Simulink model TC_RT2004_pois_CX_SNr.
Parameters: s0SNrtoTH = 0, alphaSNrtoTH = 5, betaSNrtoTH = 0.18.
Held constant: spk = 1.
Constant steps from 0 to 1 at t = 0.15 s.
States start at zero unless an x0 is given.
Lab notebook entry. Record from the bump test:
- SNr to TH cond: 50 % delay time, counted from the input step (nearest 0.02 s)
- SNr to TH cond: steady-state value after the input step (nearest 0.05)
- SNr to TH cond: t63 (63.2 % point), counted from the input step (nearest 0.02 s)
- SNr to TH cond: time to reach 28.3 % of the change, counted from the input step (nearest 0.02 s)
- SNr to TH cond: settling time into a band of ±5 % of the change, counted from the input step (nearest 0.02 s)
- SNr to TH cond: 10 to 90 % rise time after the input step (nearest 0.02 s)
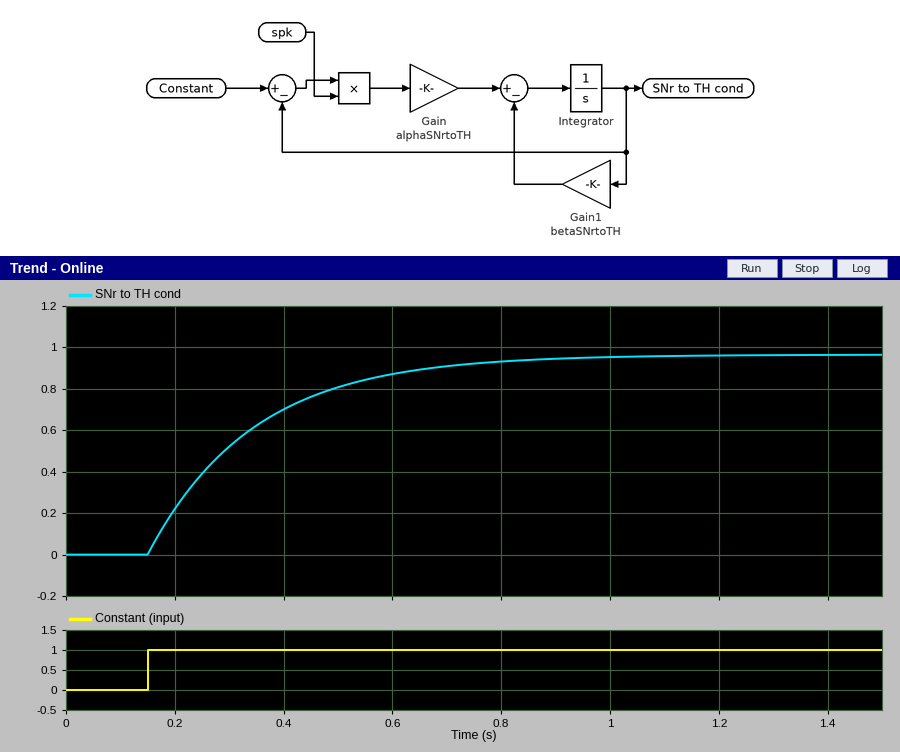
0.14 s
0.95
0.20 s
0.06 s
0.58 s
0.42 s
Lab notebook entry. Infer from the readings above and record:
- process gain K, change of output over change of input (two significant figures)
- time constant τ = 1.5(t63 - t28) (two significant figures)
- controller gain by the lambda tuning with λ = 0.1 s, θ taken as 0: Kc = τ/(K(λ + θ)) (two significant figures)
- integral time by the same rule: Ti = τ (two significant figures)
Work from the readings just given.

0.95
0.21 s
2.2
0.21 s
